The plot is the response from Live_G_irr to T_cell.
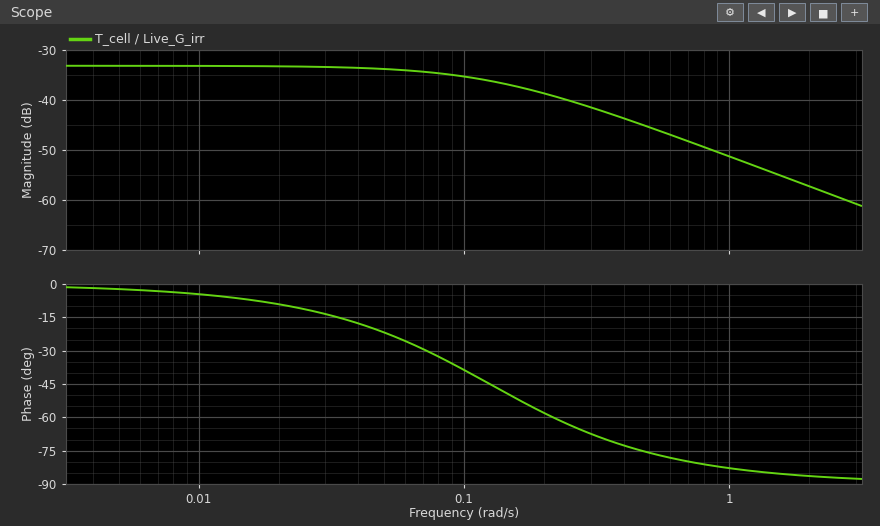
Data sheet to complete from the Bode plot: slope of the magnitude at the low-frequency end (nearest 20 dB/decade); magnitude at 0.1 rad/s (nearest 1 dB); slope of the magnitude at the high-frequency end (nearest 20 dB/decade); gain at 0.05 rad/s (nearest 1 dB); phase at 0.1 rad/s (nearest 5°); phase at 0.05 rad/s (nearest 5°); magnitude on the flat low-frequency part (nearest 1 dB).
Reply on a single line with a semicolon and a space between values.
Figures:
0 dB/decade; -35 dB; -20 dB/decade; -34 dB; -40°; -20°; -33 dB
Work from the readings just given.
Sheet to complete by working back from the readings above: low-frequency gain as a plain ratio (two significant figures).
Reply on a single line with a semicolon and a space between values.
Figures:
0.022
